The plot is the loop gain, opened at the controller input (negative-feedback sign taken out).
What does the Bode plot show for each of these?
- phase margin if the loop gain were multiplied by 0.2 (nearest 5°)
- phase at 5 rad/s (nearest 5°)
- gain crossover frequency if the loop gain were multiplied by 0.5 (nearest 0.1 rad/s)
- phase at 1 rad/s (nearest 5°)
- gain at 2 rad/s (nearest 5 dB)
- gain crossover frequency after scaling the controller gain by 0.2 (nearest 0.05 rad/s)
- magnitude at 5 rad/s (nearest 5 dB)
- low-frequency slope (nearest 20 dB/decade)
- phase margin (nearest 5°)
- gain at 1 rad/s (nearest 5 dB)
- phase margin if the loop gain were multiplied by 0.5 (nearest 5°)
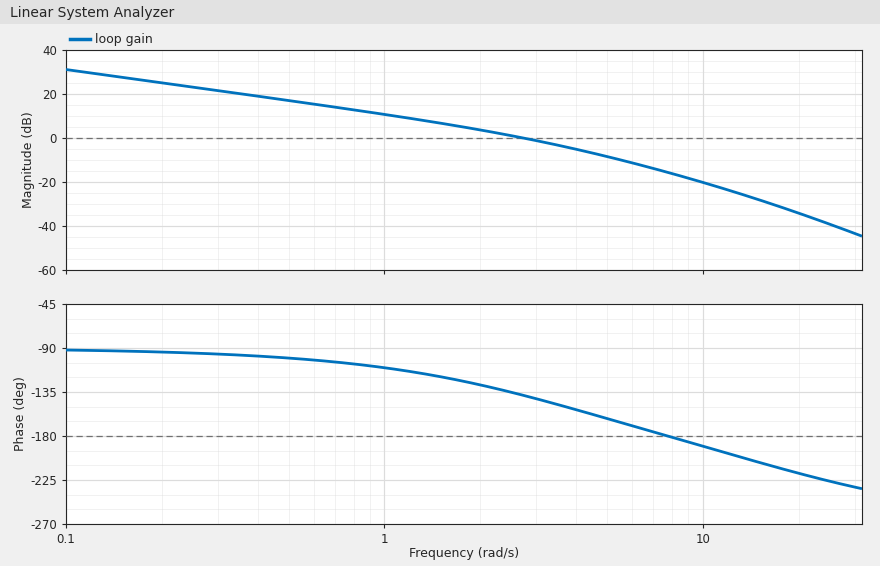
75°
-160°
1.6 rad/s
-110°
5 dB
0.70 rad/s
-10 dB
-20 dB/decade
40°
10 dB
60°
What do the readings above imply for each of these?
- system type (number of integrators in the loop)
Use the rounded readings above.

1
